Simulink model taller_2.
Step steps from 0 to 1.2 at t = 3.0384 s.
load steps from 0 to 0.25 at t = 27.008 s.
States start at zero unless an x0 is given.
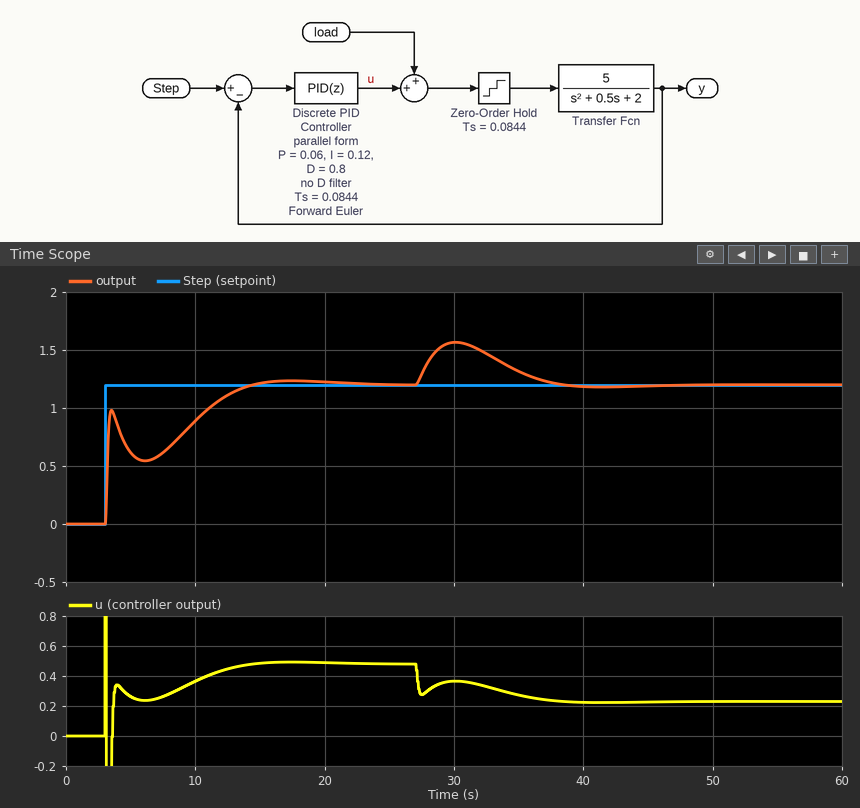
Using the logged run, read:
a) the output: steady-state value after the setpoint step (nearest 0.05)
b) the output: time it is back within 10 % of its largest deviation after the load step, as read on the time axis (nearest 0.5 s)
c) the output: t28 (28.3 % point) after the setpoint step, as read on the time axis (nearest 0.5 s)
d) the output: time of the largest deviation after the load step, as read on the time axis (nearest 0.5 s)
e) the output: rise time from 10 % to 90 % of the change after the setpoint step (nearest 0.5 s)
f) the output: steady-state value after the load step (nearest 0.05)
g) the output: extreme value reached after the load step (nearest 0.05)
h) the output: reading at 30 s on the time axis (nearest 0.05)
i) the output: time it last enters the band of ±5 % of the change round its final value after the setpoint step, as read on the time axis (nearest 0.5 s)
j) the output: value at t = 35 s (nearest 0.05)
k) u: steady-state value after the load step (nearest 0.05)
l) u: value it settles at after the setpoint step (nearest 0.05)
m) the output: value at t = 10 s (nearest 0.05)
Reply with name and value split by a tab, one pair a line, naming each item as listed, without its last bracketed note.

the output: steady-state value after the setpoint step	1.20
the output: time it is back within 10 % of its largest deviation after the load step, as read on the time axis	37.0 s
the output: t28 (28.3 % point) after the setpoint step, as read on the time axis	3.0 s
the output: time of the largest deviation after the load step, as read on the time axis	30.0 s
the output: rise time from 10 % to 90 % of the change after the setpoint step	9.0 s
the output: steady-state value after the load step	1.20
the output: extreme value reached after the load step	1.55
the output: reading at 30 s on the time axis	1.55
the output: time it last enters the band of ±5 % of the change round its final value after the setpoint step, as read on the time axis	13.0 s
the output: value at t = 35 s	1.30
u: steady-state value after the load step	0.25
u: value it settles at after the setpoint step	0.50
the output: value at t = 10 s	0.90
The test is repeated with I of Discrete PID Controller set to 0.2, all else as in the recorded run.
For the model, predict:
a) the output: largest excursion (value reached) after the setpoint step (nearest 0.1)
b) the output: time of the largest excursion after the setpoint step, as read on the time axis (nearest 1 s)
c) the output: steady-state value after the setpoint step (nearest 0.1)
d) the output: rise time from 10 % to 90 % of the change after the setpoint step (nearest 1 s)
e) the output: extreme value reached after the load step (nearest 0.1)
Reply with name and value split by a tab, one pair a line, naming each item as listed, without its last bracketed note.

the output: largest excursion (value reached) after the setpoint step	1.3
the output: time of the largest excursion after the setpoint step, as read on the time axis	13 s
the output: steady-state value after the setpoint step	1.2
the output: rise time from 10 % to 90 % of the change after the setpoint step	6 s
the output: extreme value reached after the load step	1.5
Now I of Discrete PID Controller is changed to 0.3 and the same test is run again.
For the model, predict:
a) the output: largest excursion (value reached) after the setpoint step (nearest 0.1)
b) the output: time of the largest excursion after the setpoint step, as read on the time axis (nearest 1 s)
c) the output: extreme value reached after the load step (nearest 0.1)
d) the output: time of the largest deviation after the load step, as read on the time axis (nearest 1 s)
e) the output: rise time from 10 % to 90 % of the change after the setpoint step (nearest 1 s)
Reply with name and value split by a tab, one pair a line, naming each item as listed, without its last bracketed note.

the output: largest excursion (value reached) after the setpoint step	1.3
the output: time of the largest excursion after the setpoint step, as read on the time axis	11 s
the output: extreme value reached after the load step	1.5
the output: time of the largest deviation after the load step, as read on the time axis	29 s
the output: rise time from 10 % to 90 % of the change after the setpoint step	5 s
